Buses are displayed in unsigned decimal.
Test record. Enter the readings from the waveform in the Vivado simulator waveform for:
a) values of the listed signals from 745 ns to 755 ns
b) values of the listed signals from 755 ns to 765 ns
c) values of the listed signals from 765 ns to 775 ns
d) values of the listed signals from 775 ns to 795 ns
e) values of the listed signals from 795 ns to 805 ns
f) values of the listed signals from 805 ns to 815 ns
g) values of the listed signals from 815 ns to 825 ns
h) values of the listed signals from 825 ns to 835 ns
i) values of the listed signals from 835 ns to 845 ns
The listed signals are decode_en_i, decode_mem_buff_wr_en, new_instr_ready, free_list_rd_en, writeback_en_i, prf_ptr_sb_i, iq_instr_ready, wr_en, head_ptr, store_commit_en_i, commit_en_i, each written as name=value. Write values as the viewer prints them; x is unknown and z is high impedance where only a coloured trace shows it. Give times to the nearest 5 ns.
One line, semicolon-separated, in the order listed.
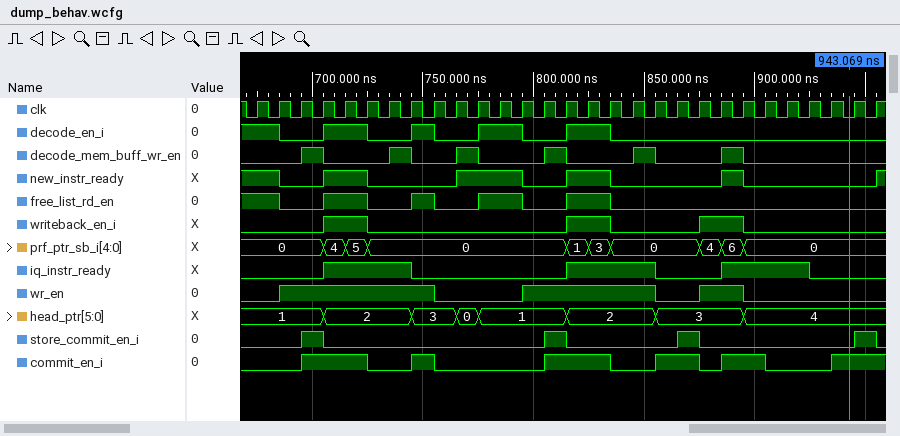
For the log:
decode_en_i=1, decode_mem_buff_wr_en=0, new_instr_ready=0, free_list_rd_en=1, writeback_en_i=0, prf_ptr_sb_i=0, iq_instr_ready=0, wr_en=1, head_ptr=3, store_commit_en_i=0, commit_en_i=1; decode_en_i=0, decode_mem_buff_wr_en=0, new_instr_ready=0, free_list_rd_en=0, writeback_en_i=0, prf_ptr_sb_i=0, iq_instr_ready=0, wr_en=0, head_ptr=3, store_commit_en_i=0, commit_en_i=0; decode_en_i=0, decode_mem_buff_wr_en=1, new_instr_ready=1, free_list_rd_en=0, writeback_en_i=0, prf_ptr_sb_i=0, iq_instr_ready=0, wr_en=0, head_ptr=0, store_commit_en_i=0, commit_en_i=0; decode_en_i=1, decode_mem_buff_wr_en=0, new_instr_ready=1, free_list_rd_en=1, writeback_en_i=0, prf_ptr_sb_i=0, iq_instr_ready=0, wr_en=0, head_ptr=1, store_commit_en_i=0, commit_en_i=0; decode_en_i=0, decode_mem_buff_wr_en=0, new_instr_ready=0, free_list_rd_en=0, writeback_en_i=0, prf_ptr_sb_i=0, iq_instr_ready=0, wr_en=1, head_ptr=1, store_commit_en_i=0, commit_en_i=0; decode_en_i=0, decode_mem_buff_wr_en=1, new_instr_ready=0, free_list_rd_en=0, writeback_en_i=0, prf_ptr_sb_i=0, iq_instr_ready=0, wr_en=1, head_ptr=1, store_commit_en_i=1, commit_en_i=1; decode_en_i=1, decode_mem_buff_wr_en=0, new_instr_ready=1, free_list_rd_en=1, writeback_en_i=1, prf_ptr_sb_i=1, iq_instr_ready=1, wr_en=1, head_ptr=2, store_commit_en_i=0, commit_en_i=1; decode_en_i=1, decode_mem_buff_wr_en=0, new_instr_ready=1, free_list_rd_en=1, writeback_en_i=1, prf_ptr_sb_i=3, iq_instr_ready=1, wr_en=1, head_ptr=2, store_commit_en_i=0, commit_en_i=1; decode_en_i=0, decode_mem_buff_wr_en=0, new_instr_ready=0, free_list_rd_en=0, writeback_en_i=0, prf_ptr_sb_i=0, iq_instr_ready=1, wr_en=1, head_ptr=2, store_commit_en_i=0, commit_en_i=0
